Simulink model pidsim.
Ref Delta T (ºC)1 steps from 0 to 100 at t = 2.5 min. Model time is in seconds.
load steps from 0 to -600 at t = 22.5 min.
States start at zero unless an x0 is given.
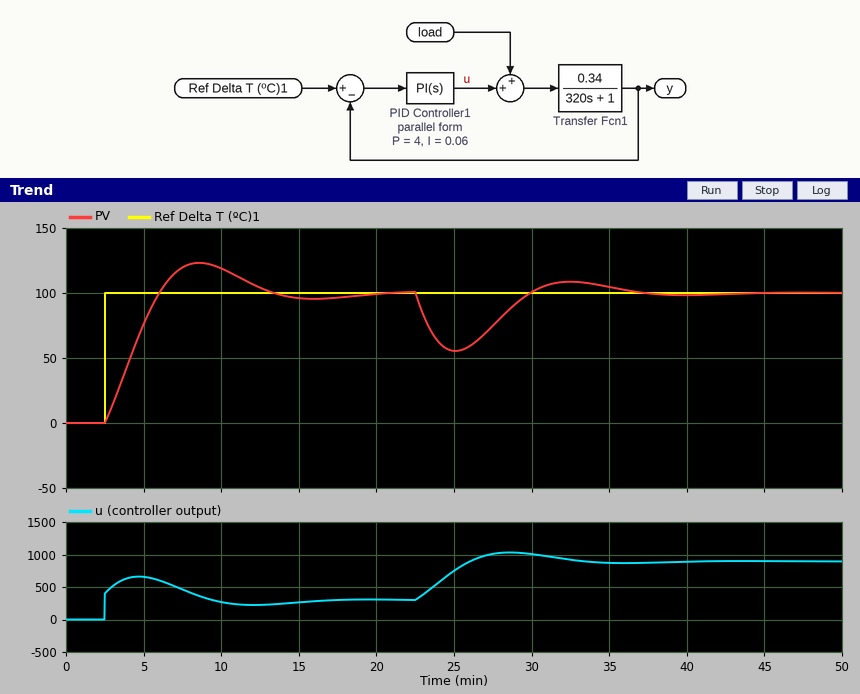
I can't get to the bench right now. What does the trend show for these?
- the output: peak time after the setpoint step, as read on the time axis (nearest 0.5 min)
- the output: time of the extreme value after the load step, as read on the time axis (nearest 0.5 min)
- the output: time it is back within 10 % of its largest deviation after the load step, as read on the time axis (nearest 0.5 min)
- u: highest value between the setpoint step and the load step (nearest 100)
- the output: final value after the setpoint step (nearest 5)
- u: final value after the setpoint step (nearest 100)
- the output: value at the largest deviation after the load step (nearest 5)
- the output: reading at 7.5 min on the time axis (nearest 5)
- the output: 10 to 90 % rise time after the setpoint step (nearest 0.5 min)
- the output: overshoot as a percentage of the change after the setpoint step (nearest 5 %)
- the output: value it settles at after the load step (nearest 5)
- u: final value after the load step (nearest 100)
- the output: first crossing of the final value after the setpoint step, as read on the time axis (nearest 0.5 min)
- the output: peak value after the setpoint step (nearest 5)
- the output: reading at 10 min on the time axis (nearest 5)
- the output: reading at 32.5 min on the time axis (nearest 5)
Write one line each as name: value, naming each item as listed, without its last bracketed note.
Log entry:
the output: peak time after the setpoint step, as read on the time axis: 8.5 min
the output: time of the extreme value after the load step, as read on the time axis: 25.0 min
the output: time it is back within 10 % of its largest deviation after the load step, as read on the time axis: 35.0 min
u: highest value between the setpoint step and the load step: 700
the output: final value after the setpoint step: 100
u: final value after the setpoint step: 300
the output: value at the largest deviation after the load step: 55
the output: reading at 7.5 min on the time axis: 120
the output: 10 to 90 % rise time after the setpoint step: 2.5 min
the output: overshoot as a percentage of the change after the setpoint step: 25 %
the output: value it settles at after the load step: 100
u: final value after the load step: 900
the output: first crossing of the final value after the setpoint step, as read on the time axis: 6.0 min
the output: peak value after the setpoint step: 125
the output: reading at 10 min on the time axis: 120
the output: reading at 32.5 min on the time axis: 110
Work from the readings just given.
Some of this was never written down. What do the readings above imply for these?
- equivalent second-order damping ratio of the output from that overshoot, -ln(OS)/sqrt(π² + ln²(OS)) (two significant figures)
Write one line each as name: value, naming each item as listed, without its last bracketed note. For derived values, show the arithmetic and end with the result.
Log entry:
equivalent second-order damping ratio of the output from that overshoot, -ln(OS)/sqrt(π² + ln²(OS)): ln(0.25) = -1.386; 1.386 / sqrt(9.870 + 1.922) = 0.40
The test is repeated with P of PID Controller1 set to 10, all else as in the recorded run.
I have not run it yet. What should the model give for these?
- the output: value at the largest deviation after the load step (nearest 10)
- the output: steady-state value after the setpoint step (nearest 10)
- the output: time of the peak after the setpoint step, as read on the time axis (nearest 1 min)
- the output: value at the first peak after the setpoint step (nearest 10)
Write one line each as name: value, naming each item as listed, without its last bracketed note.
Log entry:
the output: value at the largest deviation after the load step: 70
the output: steady-state value after the setpoint step: 100
the output: time of the peak after the setpoint step, as read on the time axis: 8 min
the output: value at the first peak after the setpoint step: 110
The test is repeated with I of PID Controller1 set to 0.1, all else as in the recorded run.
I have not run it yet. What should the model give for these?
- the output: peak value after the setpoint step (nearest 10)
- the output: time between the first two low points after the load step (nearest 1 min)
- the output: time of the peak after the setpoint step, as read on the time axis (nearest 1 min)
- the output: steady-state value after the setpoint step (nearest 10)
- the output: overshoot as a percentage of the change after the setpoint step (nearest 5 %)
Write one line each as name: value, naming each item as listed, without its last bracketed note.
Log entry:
the output: peak value after the setpoint step: 130
the output: time between the first two low points after the load step: 11 min
the output: time of the peak after the setpoint step, as read on the time axis: 7 min
the output: steady-state value after the setpoint step: 100
the output: overshoot as a percentage of the change after the setpoint step: 35 %
